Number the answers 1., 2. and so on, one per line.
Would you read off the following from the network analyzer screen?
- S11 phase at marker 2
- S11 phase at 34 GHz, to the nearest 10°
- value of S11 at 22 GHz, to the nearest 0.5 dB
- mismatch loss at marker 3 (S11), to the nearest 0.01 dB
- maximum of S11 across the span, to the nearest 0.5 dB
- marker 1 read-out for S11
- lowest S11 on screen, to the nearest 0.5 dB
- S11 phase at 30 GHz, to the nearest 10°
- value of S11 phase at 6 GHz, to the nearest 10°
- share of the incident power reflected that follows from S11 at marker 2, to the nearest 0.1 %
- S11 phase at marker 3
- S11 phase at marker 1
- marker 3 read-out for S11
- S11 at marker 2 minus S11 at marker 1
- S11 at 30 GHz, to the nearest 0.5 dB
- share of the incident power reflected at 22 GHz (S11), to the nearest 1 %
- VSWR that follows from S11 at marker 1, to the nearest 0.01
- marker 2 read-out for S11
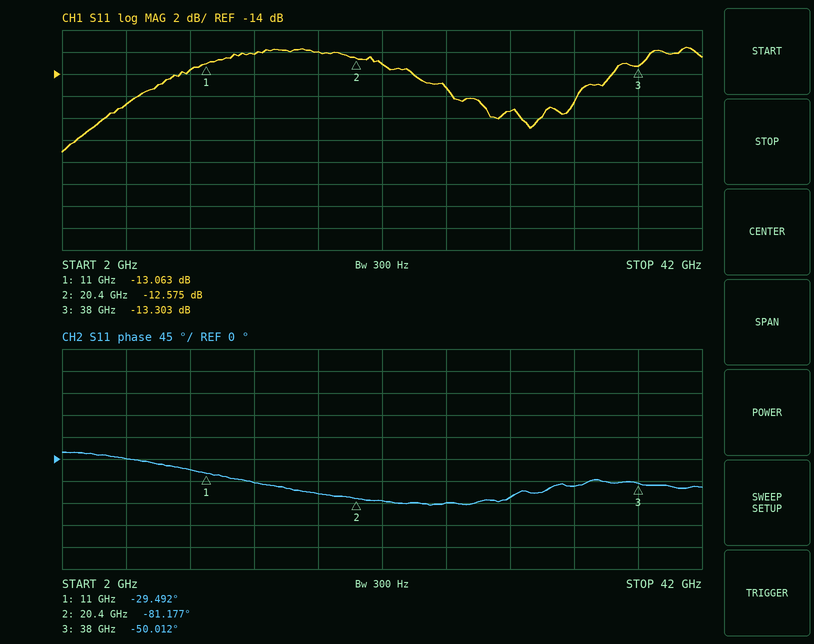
1. -81.177°
2. -60°
3. -13.0 dB
4. 0.21 dB
5. -11.5 dB
6. -13.063 dB
7. -21.0 dB
8. -80°
9. 0°
10. 5.5 %
11. -50.012°
12. -29.492°
13. -13.303 dB
14. 0.488 dB
15. -17.5 dB
16. 5 %
17. 1.57
18. -12.575 dB
